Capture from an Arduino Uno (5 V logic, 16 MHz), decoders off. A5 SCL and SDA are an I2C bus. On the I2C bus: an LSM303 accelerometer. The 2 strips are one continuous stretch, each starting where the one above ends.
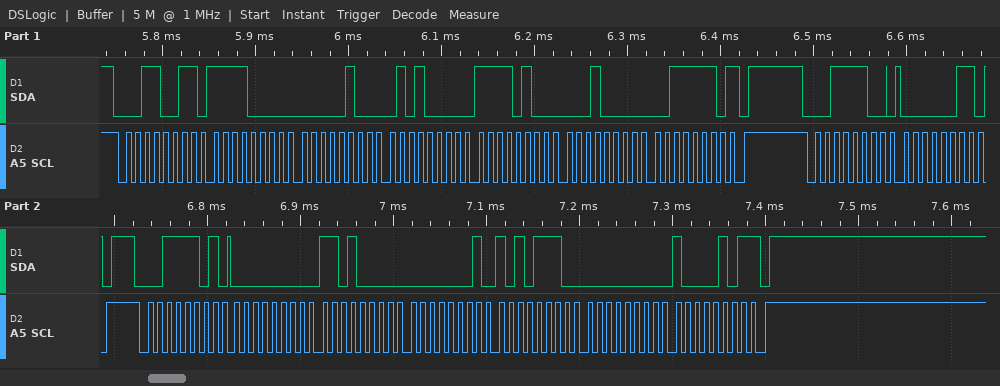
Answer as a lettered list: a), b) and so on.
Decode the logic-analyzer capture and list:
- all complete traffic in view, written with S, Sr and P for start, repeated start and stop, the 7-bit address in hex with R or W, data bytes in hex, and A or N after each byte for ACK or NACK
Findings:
a) S 19R A F0 A 04 A 50 A F4 A 10 A 3E N P S 1EW A 03 A P S 1ER A 00 A D0 A 01 A AE A 00 A 85 N P
